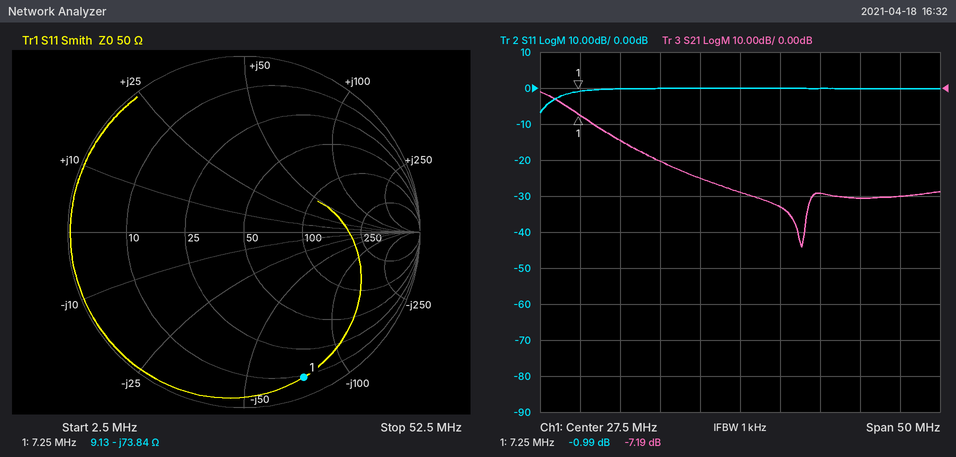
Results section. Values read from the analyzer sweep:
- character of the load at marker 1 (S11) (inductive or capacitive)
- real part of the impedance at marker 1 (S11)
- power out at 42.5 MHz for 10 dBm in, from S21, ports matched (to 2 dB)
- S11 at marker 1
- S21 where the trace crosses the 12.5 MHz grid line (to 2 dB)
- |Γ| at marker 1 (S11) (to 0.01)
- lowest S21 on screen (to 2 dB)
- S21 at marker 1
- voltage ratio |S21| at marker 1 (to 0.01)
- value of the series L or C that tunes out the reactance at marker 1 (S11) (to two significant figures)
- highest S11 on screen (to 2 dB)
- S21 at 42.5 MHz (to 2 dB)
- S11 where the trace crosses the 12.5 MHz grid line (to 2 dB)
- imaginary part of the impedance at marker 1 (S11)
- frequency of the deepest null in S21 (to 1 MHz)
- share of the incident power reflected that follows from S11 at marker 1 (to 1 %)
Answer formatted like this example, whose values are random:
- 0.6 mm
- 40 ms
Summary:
- capacitive
- 9.13 Ω
- -20 dBm
- -0.99 dB
- -14 dB
- 0.89
- -44 dB
- -7.19 dB
- 0.44
- 1.6 µH
- 0 dB
- -30 dB
- 0 dB
- -73.84 Ω
- 35 MHz
- 80 %
